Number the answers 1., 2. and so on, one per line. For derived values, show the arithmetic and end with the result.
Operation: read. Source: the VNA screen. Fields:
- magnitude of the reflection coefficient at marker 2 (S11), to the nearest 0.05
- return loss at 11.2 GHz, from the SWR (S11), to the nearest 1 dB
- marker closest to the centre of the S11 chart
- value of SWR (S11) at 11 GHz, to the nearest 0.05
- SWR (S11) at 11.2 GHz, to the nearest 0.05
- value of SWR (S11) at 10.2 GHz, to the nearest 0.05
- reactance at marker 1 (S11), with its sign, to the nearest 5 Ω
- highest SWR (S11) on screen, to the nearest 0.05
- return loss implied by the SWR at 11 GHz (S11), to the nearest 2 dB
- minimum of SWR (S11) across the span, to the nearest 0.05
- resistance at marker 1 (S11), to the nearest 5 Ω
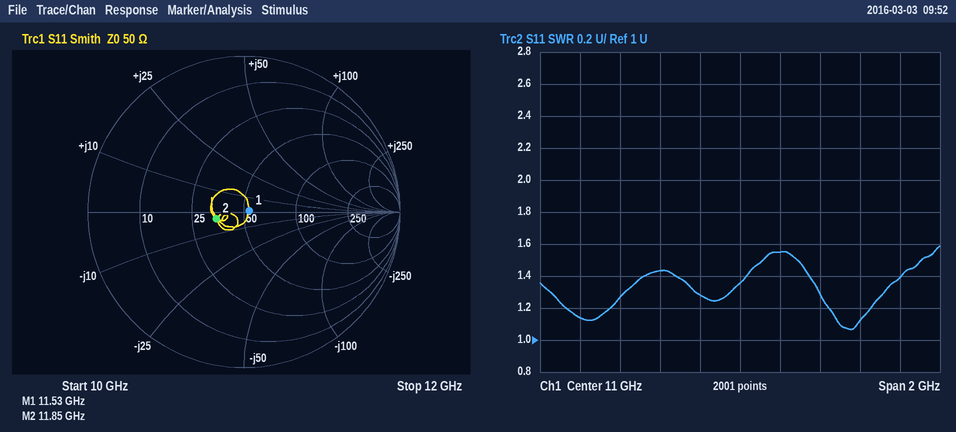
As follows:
1. 0.20
2. −20 log10((1.55 − 1)/(1.55 + 1)) ≈ 13 dB
3. marker 1
4. 1.35
5. 1.55
6. 1.15
7. 0 Ω
8. 1.60
9. −20 log10((1.35 − 1)/(1.35 + 1)) ≈ 16 dB
10. 1.05
11. 55 Ω
